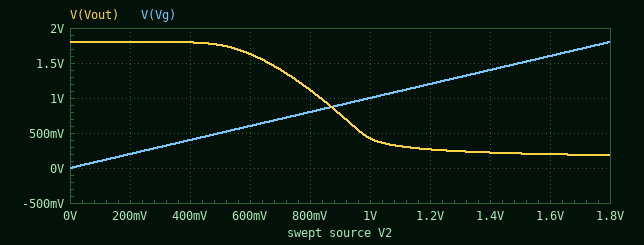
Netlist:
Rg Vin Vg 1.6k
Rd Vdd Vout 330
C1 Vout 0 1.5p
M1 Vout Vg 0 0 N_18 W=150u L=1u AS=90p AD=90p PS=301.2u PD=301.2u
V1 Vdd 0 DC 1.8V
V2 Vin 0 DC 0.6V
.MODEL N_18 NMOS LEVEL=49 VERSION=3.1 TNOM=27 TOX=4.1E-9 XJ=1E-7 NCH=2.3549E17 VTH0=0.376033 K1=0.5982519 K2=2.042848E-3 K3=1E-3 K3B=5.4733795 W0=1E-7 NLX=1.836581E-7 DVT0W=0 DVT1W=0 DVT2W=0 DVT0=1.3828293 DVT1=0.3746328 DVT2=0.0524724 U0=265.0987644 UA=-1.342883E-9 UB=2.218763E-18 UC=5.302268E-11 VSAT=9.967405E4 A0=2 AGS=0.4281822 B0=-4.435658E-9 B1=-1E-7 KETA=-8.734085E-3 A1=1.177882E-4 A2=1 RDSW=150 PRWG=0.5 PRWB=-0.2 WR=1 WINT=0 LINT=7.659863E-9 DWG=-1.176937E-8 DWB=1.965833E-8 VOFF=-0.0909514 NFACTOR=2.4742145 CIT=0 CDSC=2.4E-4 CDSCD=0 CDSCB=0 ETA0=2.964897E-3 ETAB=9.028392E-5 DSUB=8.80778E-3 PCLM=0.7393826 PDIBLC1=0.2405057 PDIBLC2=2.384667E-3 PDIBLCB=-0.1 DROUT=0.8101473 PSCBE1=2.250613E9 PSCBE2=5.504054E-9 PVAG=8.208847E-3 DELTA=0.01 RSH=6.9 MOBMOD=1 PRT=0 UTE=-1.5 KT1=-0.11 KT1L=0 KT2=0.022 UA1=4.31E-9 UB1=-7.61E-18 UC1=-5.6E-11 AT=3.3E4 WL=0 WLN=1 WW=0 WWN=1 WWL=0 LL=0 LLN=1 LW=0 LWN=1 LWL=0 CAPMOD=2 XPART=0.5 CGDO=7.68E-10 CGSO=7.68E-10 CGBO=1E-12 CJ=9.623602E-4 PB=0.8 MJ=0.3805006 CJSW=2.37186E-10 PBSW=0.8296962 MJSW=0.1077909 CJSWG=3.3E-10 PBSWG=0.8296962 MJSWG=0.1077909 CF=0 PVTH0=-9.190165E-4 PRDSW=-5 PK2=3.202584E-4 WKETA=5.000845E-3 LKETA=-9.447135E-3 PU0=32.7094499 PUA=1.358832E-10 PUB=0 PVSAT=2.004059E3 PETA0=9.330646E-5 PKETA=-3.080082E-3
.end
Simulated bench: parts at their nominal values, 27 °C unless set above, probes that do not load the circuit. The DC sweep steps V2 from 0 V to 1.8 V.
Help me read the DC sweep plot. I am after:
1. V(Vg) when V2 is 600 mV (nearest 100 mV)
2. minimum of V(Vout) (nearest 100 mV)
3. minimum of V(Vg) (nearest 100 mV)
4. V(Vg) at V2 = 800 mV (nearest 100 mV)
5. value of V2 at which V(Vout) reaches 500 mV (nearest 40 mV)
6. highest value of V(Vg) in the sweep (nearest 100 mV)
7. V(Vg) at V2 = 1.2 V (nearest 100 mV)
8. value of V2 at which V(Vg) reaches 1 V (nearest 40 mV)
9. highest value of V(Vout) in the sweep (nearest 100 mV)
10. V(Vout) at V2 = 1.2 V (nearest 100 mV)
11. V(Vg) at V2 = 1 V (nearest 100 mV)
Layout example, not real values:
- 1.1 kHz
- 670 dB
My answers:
- 600 mV
- 200 mV
- 0 V
- 800 mV
- 960 mV
- 1.8 V
- 1.2 V
- 1.00 V
- 1.8 V
- 300 mV
- 1.0 V
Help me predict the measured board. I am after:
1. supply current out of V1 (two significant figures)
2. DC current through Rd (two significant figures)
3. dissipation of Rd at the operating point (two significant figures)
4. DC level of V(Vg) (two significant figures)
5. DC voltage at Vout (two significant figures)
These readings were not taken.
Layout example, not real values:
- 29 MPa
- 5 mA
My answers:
- 520 µA
- 520 µA
- 88 µW
- 600 mV
- 1.6 V
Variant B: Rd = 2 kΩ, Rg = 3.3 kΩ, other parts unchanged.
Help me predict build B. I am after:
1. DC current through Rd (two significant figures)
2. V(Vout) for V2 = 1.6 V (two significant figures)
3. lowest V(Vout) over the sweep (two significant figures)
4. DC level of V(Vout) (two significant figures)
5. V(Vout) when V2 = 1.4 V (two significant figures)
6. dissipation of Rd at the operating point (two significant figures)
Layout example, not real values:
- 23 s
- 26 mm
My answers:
- 480 µA
- 34 mV
- 32 mV
- 840 mV
- 37 mV
- 460 µW
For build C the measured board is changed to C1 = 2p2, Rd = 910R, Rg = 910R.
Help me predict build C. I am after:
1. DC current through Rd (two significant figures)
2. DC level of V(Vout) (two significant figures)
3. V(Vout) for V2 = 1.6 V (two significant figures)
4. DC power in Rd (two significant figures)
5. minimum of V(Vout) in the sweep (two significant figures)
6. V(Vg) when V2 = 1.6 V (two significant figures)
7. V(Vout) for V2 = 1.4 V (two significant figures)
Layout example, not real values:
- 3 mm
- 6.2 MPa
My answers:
- 500 µA
- 1.3 V
- 73 mV
- 230 µW
- 69 mV
- 1.6 V
- 81 mV
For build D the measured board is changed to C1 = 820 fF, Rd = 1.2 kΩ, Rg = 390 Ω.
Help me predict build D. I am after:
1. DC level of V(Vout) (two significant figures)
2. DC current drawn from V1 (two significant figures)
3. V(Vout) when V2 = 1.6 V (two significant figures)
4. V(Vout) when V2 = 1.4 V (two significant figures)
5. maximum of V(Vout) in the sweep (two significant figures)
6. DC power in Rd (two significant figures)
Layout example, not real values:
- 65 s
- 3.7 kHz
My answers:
- 1.2 V
- 500 µA
- 56 mV
- 61 mV
- 1.8 V
- 300 µW
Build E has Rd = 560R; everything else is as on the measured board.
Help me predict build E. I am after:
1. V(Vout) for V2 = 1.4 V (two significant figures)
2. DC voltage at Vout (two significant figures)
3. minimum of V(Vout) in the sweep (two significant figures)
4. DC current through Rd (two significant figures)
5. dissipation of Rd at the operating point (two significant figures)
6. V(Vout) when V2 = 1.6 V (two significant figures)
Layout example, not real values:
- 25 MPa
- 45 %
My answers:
- 130 mV
- 1.5 V
- 110 mV
- 510 µA
- 150 µW
- 120 mV
